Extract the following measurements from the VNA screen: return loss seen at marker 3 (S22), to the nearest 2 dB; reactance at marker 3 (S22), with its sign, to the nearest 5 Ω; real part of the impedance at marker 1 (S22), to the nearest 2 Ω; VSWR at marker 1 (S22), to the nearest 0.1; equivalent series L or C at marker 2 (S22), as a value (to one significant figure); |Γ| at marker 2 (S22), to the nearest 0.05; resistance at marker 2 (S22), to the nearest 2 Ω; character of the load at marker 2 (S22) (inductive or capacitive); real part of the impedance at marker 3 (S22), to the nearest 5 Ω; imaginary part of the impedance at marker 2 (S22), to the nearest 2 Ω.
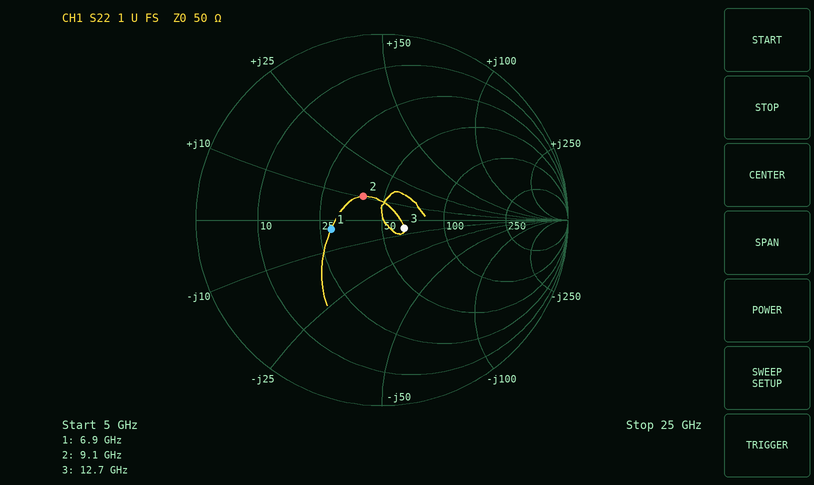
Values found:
18 dB
-5 Ω
28 Ω
1.8
200 pH
0.15
40 Ω
inductive
65 Ω
+10 Ω
